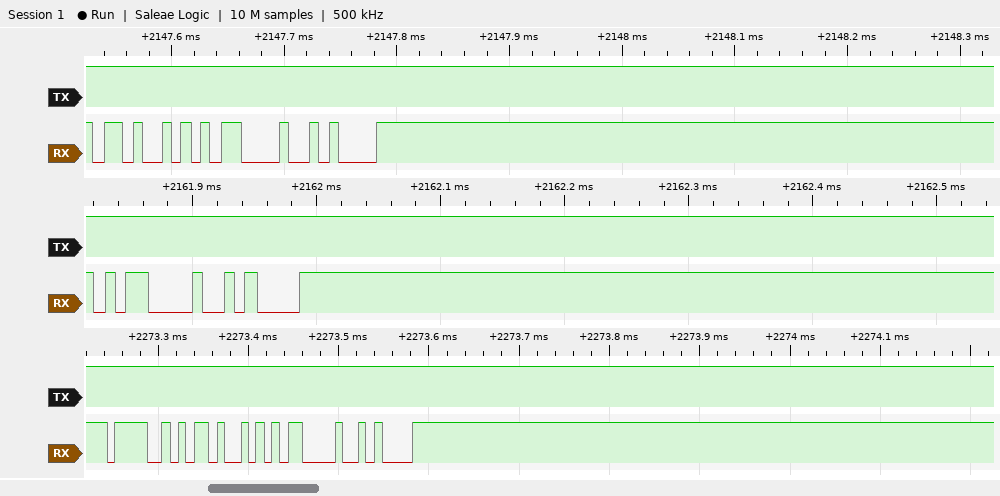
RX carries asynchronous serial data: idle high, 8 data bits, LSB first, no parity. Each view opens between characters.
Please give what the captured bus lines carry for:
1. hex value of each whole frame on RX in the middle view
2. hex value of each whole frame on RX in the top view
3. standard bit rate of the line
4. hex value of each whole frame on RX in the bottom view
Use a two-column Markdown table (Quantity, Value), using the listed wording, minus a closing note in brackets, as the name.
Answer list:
| Quantity | Value |
|---|---|
| hex value of each whole frame on RX in the middle view | 0D, 0A |
| hex value of each whole frame on RX in the top view | 4B, 0D, 0A |
| standard bit rate of the line | 115200 baud |
| hex value of each whole frame on RX in the bottom view | 4F, 4B, 0D, 0A |
